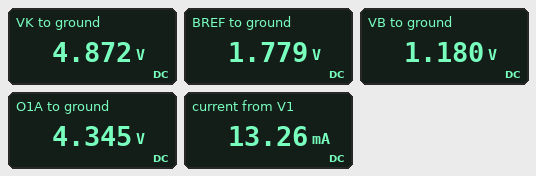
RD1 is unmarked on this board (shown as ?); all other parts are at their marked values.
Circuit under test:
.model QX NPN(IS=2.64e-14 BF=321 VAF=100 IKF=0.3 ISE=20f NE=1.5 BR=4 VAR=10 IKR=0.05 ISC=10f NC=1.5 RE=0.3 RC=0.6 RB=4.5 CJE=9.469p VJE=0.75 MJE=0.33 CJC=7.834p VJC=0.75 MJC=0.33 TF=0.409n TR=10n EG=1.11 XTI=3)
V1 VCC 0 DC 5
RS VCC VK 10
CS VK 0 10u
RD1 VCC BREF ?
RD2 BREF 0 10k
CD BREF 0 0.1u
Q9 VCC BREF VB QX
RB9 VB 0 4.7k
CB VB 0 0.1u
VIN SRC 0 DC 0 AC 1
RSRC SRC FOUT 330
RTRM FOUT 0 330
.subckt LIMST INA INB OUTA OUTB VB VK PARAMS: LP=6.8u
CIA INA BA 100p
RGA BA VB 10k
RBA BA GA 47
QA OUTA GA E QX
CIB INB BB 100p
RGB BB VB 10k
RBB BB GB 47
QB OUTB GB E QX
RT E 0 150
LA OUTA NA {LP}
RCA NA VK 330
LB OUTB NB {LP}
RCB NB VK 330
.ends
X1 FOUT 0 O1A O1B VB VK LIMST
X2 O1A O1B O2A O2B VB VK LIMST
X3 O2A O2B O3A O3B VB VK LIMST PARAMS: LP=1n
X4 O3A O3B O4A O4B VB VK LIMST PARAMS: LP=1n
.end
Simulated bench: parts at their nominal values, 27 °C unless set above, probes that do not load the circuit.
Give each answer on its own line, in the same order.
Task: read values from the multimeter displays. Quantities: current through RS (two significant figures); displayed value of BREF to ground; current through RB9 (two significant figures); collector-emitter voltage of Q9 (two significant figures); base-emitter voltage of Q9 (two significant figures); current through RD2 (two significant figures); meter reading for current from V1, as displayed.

13 mA
1.779 V
250 µA
3.8 V
600 mV
180 µA
13.26 mA
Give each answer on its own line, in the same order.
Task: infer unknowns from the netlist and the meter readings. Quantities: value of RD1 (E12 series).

18 kΩ
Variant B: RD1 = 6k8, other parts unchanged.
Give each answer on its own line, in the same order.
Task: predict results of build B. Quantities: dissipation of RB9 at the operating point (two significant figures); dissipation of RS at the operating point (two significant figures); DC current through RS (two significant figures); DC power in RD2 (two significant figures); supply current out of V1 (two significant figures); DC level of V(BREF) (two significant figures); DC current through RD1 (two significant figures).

1.2 mW
16 mW
40 mA
880 µW
41 mA
3.0 V
300 µA
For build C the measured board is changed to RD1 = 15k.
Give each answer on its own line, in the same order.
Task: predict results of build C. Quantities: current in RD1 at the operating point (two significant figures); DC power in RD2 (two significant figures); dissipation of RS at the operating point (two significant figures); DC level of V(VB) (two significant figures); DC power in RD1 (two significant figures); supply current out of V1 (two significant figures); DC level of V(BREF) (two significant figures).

200 µA
400 µW
3.1 mW
1.4 V
600 µW
18 mA
2.0 V
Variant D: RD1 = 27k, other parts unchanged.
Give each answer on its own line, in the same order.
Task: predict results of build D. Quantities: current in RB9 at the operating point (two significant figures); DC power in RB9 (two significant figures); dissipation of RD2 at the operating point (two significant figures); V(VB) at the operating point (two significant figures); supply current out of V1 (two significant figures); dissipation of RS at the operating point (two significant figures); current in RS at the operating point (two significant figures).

160 µA
120 µW
180 µW
760 mV
3.9 mA
130 µW
3.6 mA
